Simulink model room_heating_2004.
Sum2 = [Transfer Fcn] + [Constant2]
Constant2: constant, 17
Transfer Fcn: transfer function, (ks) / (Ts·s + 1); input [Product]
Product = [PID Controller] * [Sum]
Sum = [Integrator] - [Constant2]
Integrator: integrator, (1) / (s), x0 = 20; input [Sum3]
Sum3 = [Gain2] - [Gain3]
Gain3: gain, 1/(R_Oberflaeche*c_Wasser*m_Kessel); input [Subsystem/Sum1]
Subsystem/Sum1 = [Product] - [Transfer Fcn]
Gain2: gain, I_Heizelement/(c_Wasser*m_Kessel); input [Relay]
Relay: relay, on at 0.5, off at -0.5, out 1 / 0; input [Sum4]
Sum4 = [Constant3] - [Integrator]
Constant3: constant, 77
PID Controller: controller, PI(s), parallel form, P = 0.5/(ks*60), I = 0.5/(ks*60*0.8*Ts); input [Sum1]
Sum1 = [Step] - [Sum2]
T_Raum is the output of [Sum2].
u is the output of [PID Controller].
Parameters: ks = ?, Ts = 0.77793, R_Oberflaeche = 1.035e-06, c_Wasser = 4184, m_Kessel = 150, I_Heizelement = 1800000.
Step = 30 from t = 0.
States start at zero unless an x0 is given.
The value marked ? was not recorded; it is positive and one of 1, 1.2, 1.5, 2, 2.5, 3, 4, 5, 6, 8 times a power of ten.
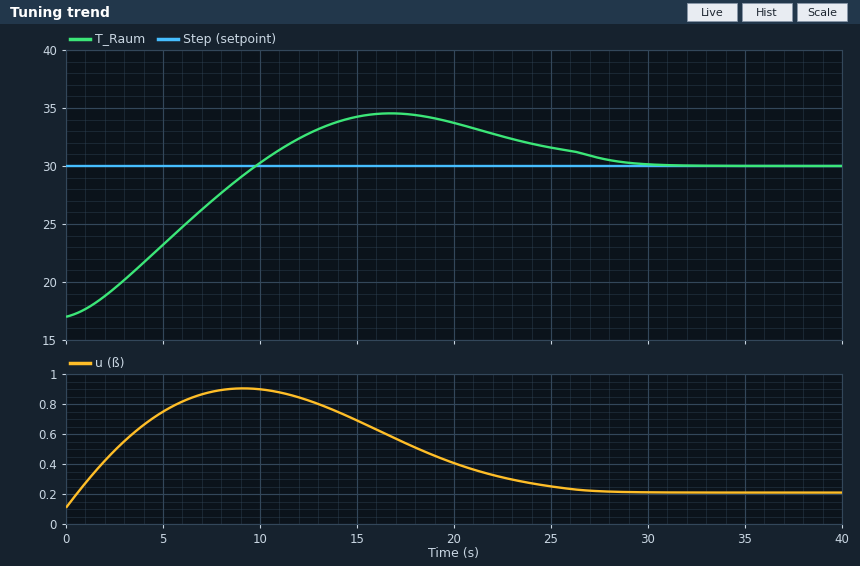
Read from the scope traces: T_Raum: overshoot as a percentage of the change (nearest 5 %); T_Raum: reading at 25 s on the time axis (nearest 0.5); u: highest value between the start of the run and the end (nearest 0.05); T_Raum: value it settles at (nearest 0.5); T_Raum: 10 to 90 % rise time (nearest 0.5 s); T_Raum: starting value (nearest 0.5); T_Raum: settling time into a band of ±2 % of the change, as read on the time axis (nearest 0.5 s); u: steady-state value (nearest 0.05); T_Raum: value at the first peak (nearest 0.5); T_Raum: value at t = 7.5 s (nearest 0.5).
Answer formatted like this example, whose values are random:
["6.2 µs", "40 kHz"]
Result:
["35 %", "31.5", "0.90", "30.0", "7.0 s", "17.0", "29.0 s", "0.20", "34.5", "27.0"]
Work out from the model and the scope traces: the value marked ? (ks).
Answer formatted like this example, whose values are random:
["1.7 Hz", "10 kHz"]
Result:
["1"]
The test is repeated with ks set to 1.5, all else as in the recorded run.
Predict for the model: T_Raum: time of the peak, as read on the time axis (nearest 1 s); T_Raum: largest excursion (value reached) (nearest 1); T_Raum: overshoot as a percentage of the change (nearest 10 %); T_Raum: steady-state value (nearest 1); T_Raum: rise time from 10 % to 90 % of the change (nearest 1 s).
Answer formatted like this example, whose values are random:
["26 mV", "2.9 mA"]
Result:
["9 s", "38", "60 %", "30", "4 s"]
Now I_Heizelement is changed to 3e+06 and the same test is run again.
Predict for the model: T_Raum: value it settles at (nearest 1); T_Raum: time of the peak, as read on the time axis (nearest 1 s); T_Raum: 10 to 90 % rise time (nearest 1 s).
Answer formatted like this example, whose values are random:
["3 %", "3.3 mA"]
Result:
["30", "12 s", "5 s"]
